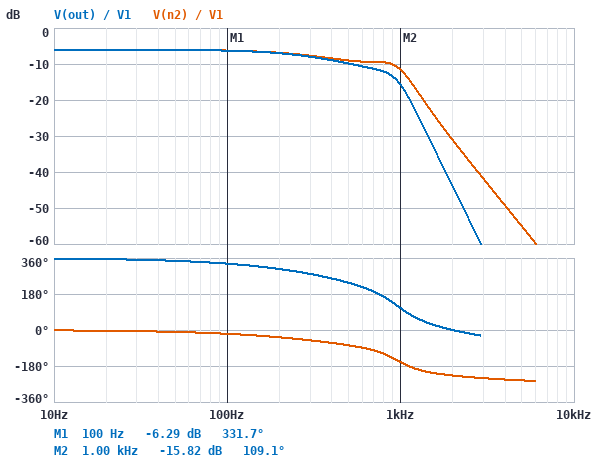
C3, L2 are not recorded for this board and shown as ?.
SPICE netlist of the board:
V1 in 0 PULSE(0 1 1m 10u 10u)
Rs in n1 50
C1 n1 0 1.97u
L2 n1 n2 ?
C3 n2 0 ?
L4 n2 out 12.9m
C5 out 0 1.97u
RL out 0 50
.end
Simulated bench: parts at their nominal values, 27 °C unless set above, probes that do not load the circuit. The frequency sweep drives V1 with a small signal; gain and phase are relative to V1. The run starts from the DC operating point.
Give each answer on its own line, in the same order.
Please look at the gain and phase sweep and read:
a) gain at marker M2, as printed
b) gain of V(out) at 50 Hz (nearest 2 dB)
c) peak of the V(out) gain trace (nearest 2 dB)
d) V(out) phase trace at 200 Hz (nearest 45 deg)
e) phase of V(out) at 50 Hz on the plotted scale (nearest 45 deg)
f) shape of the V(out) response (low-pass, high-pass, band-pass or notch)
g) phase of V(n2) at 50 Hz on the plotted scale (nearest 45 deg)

-15.82 dB
-6 dB
-6 dB
315 deg
360 deg
low-pass
0 deg
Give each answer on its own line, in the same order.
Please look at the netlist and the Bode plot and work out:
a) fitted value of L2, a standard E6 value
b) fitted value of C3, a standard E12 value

47 mH
3.9 µF
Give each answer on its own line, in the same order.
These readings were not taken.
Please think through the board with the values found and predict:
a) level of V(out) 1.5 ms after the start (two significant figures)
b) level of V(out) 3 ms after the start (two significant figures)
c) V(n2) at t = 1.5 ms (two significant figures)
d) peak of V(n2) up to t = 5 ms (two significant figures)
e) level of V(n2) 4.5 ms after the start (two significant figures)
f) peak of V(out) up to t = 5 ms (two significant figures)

93 mV
490 mV
290 mV
500 mV
500 mV
500 mV
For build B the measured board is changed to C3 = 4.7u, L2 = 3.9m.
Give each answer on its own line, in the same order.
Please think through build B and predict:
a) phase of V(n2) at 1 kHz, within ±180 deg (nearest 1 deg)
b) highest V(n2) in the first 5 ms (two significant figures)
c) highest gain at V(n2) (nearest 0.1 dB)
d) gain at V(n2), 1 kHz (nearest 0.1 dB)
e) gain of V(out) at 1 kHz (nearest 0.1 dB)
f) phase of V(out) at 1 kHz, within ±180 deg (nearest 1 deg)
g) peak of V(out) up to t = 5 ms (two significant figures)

-59 deg
640 mV
-3.9 dB
-4.3 dB
-8.5 dB
-149 deg
520 mV
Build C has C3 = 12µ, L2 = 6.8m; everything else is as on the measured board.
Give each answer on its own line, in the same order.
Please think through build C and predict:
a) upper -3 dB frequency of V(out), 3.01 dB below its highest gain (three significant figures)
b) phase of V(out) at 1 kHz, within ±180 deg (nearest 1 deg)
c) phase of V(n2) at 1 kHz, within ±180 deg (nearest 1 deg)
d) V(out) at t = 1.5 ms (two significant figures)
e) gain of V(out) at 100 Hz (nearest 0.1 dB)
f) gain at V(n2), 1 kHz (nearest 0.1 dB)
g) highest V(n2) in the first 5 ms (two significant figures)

671 Hz
148 deg
-122 deg
160 mV
-6.1 dB
-9.1 dB
510 mV
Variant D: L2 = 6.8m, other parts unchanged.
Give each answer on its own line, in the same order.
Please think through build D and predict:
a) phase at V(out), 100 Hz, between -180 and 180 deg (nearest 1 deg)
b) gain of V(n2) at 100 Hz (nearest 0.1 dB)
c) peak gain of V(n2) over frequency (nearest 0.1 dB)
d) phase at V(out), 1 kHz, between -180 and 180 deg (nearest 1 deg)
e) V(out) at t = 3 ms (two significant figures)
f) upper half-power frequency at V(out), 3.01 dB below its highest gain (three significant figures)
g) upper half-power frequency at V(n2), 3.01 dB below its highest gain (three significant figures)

-14 deg
-6.0 dB
-0.9 dB
-152 deg
500 mV
1.43 kHz
1.73 kHz
